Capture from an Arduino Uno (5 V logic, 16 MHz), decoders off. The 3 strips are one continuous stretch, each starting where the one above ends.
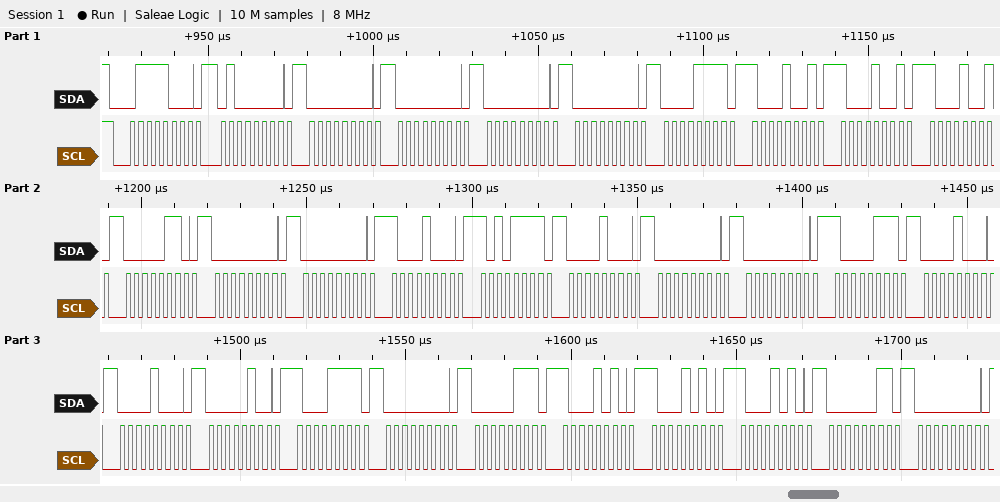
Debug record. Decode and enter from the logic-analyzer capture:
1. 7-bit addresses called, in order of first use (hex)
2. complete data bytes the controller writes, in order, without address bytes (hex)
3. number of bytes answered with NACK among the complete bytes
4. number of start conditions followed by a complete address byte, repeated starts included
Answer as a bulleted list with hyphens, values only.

- 0x3C
- 40 00 00 00 00 0F 89 89 89 06 00 00 88 AF 08 00 00 87 08 08 04 8F 00 07 8A 8A 8A 03 00
- 0
- 1
